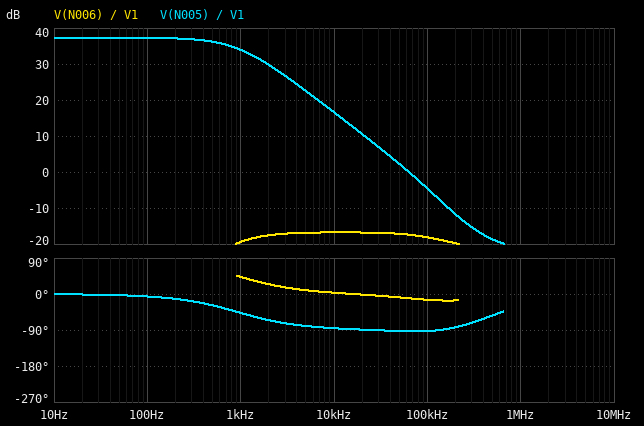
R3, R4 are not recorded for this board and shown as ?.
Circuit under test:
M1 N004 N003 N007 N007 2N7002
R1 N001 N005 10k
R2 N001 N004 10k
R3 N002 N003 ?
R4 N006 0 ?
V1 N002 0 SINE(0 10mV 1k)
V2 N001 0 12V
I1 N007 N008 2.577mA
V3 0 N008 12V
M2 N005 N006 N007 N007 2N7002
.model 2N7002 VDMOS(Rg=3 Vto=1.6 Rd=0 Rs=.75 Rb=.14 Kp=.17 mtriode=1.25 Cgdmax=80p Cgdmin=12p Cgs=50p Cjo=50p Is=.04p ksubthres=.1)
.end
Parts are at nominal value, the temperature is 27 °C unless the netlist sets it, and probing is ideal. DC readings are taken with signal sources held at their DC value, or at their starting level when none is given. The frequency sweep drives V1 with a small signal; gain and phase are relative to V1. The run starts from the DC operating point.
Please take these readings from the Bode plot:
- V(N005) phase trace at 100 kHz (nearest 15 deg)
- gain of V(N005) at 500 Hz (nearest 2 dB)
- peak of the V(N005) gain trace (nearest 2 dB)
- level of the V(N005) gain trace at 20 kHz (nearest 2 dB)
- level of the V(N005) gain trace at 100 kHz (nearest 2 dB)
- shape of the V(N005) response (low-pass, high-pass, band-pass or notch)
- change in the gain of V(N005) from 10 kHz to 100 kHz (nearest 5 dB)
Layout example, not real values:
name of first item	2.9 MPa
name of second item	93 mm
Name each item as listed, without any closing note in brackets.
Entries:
V(N005) phase trace at 100 kHz	-90 deg
gain of V(N005) at 500 Hz	36 dB
peak of the V(N005) gain trace	38 dB
level of the V(N005) gain trace at 20 kHz	10 dB
level of the V(N005) gain trace at 100 kHz	-4 dB
shape of the V(N005) response	low-pass
change in the gain of V(N005) from 10 kHz to 100 kHz	-20 dB
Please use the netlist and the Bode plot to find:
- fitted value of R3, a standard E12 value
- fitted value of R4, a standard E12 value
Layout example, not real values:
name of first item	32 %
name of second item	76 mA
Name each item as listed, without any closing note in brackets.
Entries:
fitted value of R3, a standard E12 value	27 kΩ
fitted value of R4, a standard E12 value	4.7 kΩ
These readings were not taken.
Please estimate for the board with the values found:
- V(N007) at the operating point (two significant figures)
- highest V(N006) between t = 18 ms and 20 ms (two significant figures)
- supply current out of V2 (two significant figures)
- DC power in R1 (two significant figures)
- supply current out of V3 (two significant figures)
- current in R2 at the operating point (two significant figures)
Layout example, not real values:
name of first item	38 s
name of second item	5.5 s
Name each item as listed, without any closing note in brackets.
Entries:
V(N007) at the operating point	-1.7 V
highest V(N006) between t = 18 ms and 20 ms	1.1 mV
supply current out of V2	2.6 mA
DC power in R1	17 mW
supply current out of V3	2.6 mA
current in R2 at the operating point	1.3 mA
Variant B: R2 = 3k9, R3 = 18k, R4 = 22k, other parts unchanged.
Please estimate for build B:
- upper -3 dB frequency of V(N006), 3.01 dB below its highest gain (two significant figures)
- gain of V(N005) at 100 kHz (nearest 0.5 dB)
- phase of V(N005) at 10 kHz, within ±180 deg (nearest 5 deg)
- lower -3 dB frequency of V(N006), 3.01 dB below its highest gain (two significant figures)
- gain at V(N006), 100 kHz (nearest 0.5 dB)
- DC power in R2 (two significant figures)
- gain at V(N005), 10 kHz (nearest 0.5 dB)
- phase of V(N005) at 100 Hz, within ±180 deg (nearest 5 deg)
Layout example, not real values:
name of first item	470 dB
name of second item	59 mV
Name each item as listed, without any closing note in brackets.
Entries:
upper -3 dB frequency of V(N006), 3.01 dB below its highest gain	340 kHz
gain of V(N005) at 100 kHz	2.0 dB
phase of V(N005) at 10 kHz, within ±180 deg	-80 deg
lower -3 dB frequency of V(N006), 3.01 dB below its highest gain	1.2 kHz
gain at V(N006), 100 kHz	-1.0 dB
DC power in R2	6.5 mW
gain at V(N005), 10 kHz	19.0 dB
phase of V(N005) at 100 Hz, within ±180 deg	-5 deg
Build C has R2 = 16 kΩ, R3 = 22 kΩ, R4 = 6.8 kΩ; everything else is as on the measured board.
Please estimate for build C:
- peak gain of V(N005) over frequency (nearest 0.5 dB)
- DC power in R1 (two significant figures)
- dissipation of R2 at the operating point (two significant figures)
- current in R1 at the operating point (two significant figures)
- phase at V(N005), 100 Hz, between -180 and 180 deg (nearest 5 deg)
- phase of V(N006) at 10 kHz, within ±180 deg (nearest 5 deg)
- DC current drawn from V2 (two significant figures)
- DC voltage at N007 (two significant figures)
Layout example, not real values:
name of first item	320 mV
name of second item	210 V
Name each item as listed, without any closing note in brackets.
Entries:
peak gain of V(N005) over frequency	-16.0 dB
DC power in R1	25 mW
dissipation of R2 at the operating point	16 mW
current in R1 at the operating point	1.6 mA
phase at V(N005), 100 Hz, between -180 and 180 deg	55 deg
phase of V(N006) at 10 kHz, within ±180 deg	160 deg
DC current drawn from V2	2.6 mA
DC voltage at N007	-3.9 V
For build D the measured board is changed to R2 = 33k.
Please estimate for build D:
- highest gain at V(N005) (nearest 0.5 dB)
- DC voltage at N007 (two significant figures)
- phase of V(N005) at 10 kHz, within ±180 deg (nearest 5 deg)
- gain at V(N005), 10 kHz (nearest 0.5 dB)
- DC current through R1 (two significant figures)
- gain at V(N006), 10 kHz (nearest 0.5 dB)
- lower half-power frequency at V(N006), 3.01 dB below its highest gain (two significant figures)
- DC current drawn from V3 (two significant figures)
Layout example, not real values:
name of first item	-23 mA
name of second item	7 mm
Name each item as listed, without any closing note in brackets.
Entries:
highest gain at V(N005)	-15.5 dB
DC voltage at N007	-7.8 V
phase of V(N005) at 10 kHz, within ±180 deg	70 deg
gain at V(N005), 10 kHz	-24.5 dB
DC current through R1	2.0 mA
gain at V(N006), 10 kHz	-53.0 dB
lower half-power frequency at V(N006), 3.01 dB below its highest gain	130 kHz
DC current drawn from V3	2.6 mA
